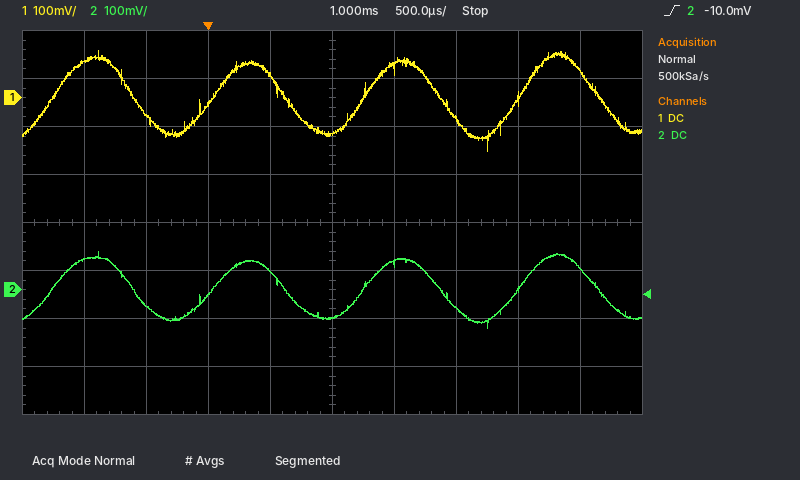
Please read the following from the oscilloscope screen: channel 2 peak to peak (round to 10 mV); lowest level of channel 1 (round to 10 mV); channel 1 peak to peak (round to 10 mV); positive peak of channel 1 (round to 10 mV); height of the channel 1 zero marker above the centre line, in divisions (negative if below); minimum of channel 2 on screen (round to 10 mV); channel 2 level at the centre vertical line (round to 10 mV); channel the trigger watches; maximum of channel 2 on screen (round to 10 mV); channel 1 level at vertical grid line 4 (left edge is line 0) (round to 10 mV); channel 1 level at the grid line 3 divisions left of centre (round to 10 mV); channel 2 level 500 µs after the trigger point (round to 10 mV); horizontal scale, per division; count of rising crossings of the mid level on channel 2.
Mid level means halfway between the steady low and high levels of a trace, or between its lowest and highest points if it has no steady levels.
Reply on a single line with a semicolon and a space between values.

160 mV; -110 mV; 210 mV; 100 mV; +2.6 div; -80 mV; -60 mV; channel 2; 80 mV; 50 mV; -30 mV; 40 mV; 500 µs; 4
